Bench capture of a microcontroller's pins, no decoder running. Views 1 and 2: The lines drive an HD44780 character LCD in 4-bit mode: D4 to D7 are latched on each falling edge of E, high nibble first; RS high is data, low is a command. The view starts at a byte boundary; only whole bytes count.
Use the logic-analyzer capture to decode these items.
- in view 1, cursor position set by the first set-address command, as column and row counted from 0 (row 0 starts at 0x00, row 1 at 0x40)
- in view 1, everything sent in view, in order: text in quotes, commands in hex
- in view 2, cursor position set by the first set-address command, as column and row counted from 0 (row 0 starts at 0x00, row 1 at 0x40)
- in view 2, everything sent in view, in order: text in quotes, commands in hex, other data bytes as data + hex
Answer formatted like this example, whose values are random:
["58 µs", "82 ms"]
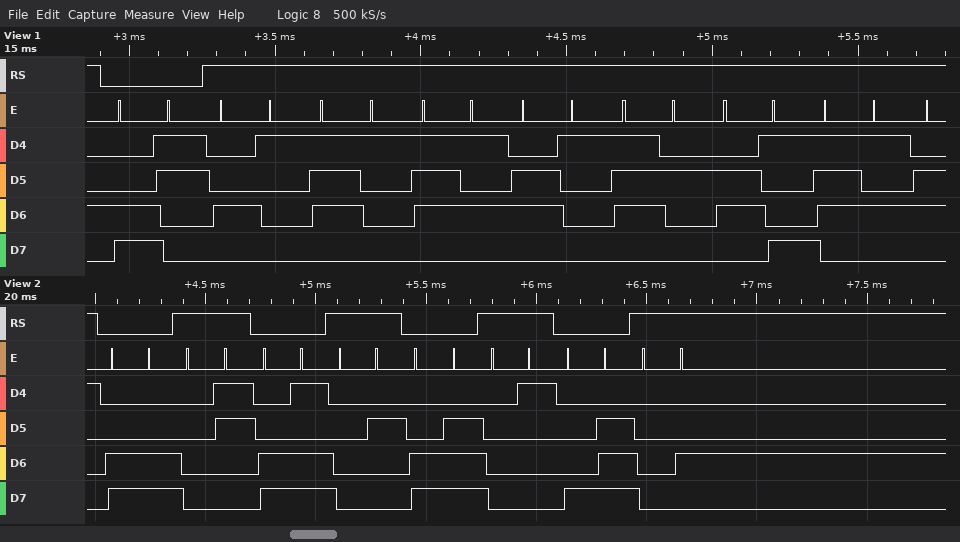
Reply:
["column 3, row 1", "0xC3 \"Aquariu\"", "column 12, row 1", "0xCC data 03 0xCD data 02 0xCE data 01 0x8E data 04"]
